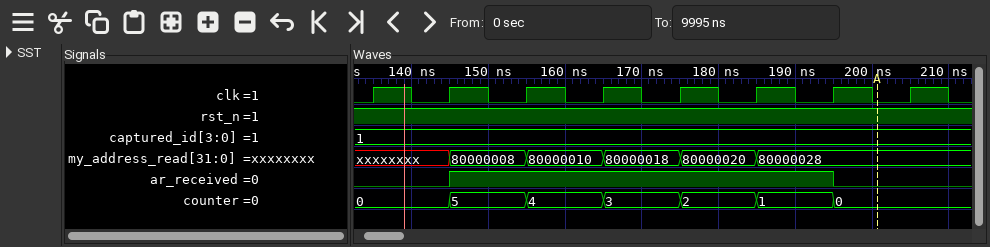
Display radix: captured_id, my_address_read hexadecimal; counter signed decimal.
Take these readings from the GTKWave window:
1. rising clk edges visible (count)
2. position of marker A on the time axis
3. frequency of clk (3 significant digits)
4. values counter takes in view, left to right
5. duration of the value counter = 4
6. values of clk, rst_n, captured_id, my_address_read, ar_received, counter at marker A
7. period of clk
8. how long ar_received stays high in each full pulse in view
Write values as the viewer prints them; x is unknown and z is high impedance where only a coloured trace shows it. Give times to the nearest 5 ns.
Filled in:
8
200 ns
100 MHz
0, 5, 4, 3, 2, 1, 0
10 ns
clk=0, rst_n=1, captured_id=1, my_address_read=80000028, ar_received=0, counter=0
10 ns
50 ns
